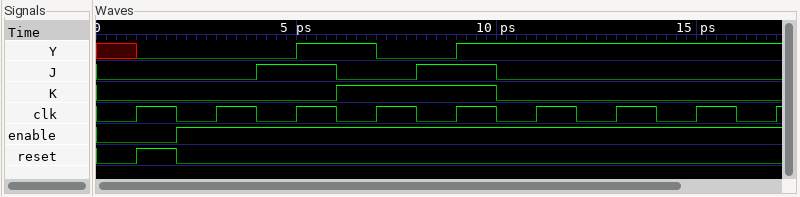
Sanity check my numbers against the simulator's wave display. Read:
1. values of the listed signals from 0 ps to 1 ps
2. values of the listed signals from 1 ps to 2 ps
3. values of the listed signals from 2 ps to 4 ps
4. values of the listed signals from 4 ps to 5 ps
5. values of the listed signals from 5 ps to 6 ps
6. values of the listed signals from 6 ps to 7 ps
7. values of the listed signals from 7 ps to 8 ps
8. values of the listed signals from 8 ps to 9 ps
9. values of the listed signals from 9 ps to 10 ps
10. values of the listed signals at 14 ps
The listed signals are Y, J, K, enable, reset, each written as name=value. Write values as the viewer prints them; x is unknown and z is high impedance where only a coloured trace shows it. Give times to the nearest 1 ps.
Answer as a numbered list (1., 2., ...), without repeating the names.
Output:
1. Y=x, J=0, K=0, enable=0, reset=0
2. Y=0, J=0, K=0, enable=0, reset=1
3. Y=0, J=0, K=0, enable=1, reset=0
4. Y=0, J=1, K=0, enable=1, reset=0
5. Y=1, J=1, K=0, enable=1, reset=0
6. Y=1, J=0, K=1, enable=1, reset=0
7. Y=0, J=0, K=1, enable=1, reset=0
8. Y=0, J=1, K=1, enable=1, reset=0
9. Y=1, J=1, K=1, enable=1, reset=0
10. Y=1, J=0, K=0, enable=1, reset=0
